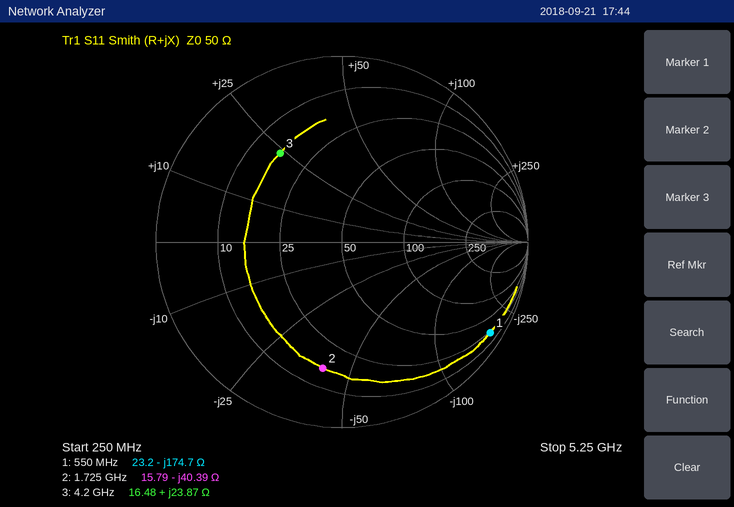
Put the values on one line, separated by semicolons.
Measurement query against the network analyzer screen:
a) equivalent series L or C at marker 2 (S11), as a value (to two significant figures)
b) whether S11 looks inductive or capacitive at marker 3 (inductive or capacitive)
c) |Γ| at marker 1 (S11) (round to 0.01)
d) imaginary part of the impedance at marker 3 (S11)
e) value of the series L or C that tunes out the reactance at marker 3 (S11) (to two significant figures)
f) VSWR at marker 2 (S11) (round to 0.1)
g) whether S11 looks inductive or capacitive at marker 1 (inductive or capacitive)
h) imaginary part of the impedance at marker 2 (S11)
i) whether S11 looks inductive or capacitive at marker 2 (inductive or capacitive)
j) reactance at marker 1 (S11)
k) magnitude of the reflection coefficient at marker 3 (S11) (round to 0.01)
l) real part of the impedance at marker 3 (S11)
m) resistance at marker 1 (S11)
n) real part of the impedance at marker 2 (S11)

2.3 pF; inductive; 0.93; +23.87 Ω; 1.6 pF; 5.4; capacitive; -40.39 Ω; capacitive; -174.7 Ω; 0.58; 16.48 Ω; 23.2 Ω; 15.79 Ω
